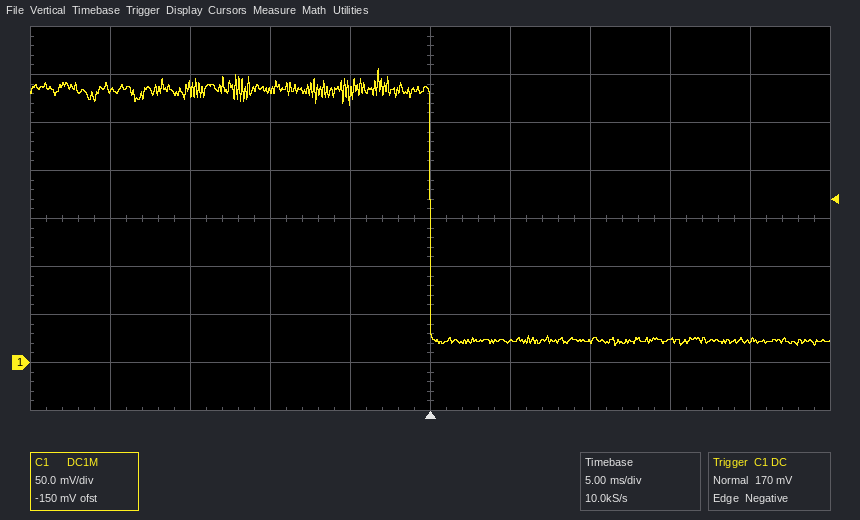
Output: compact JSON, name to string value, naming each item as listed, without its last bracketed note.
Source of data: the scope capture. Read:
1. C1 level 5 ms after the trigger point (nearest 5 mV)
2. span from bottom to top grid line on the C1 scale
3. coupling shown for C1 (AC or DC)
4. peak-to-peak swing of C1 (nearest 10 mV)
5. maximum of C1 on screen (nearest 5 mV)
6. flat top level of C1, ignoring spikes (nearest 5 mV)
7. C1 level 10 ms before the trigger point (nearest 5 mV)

{"C1 level 5 ms after the trigger point": "20 mV", "span from bottom to top grid line on the C1 scale": "400 mV", "coupling shown for C1": "DC", "peak-to-peak swing of C1": "290 mV", "maximum of C1 on screen": "305 mV", "flat top level of C1, ignoring spikes": "285 mV", "C1 level 10 ms before the trigger point": "285 mV"}
